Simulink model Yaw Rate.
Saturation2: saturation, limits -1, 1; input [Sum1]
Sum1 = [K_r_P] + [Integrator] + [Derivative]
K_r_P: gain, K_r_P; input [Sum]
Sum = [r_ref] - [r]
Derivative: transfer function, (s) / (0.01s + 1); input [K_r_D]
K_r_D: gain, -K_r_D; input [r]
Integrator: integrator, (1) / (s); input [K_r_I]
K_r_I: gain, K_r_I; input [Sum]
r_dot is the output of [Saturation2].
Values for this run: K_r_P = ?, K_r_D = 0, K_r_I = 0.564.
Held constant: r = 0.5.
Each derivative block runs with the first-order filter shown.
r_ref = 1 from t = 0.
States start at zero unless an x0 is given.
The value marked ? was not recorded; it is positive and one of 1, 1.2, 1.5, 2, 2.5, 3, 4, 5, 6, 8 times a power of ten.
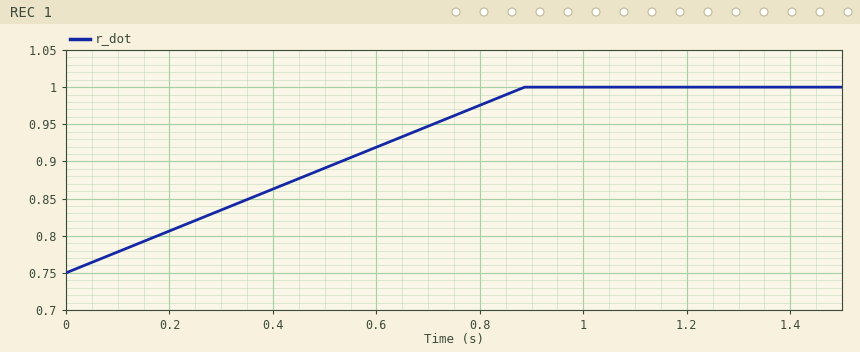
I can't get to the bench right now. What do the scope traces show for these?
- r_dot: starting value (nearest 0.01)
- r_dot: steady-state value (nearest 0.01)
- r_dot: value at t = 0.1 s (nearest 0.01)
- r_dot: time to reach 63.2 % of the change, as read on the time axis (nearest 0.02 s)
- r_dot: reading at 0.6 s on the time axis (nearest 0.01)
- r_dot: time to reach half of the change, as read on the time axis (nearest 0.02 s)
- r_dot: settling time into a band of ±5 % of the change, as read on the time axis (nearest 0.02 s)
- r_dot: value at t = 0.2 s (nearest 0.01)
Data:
0.75
1.00
0.78
0.56 s
0.92
0.44 s
0.84 s
0.81
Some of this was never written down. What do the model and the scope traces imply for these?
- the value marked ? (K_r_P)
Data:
1.5
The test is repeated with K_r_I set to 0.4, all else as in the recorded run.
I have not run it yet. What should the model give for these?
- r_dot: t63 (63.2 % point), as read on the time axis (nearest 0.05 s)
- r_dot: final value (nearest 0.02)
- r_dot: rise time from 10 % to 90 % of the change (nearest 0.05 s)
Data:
0.80 s
1.00
1.00 s
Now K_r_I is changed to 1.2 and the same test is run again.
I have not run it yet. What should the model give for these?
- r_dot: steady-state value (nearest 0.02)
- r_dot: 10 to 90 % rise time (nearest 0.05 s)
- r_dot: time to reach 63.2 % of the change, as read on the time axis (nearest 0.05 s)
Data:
1.00
0.35 s
0.25 s
